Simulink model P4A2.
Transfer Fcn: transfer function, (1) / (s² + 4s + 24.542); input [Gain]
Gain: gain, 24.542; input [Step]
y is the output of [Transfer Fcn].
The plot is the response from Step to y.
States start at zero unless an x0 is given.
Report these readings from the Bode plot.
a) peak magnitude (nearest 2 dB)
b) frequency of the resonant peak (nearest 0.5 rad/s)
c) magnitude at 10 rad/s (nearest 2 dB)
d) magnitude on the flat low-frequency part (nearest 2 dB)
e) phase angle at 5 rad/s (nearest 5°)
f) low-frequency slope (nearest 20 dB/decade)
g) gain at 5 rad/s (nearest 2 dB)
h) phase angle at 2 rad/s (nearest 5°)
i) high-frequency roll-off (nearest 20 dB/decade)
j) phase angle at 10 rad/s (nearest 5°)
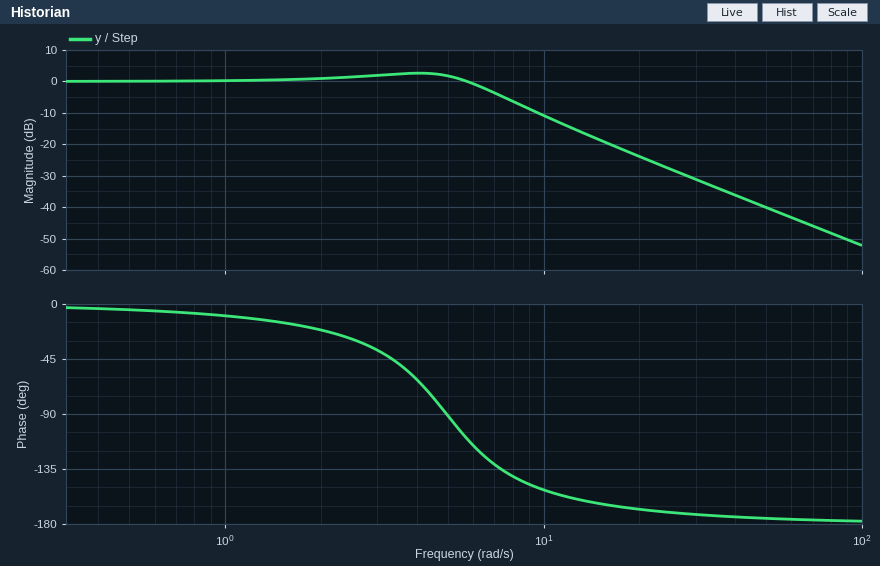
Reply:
2 dB
4.0 rad/s
-10 dB
0 dB
-90°
0 dB/decade
2 dB
-20°
-40 dB/decade
-150°
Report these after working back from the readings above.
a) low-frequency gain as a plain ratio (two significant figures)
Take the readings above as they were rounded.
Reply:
1.0
